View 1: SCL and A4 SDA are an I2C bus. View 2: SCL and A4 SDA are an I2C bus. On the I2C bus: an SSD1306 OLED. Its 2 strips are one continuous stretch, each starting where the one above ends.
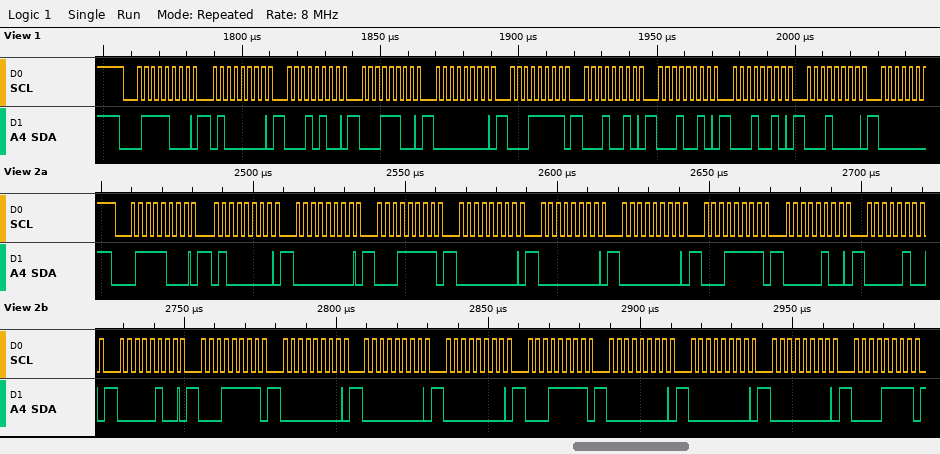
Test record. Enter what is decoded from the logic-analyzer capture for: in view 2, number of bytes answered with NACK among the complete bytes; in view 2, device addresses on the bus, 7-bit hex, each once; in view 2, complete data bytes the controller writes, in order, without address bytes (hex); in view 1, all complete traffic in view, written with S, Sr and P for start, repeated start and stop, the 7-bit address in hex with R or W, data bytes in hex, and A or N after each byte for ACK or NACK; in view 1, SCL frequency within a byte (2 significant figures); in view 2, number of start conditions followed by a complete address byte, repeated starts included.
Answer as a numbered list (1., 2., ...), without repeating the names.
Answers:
1. 0
2. 0x3C
3. 40 00 1F 00 00 00 1F 04 04 04 1F 00 00 00 1F 00 00 00 0F
4. S 3CW A 40 A 14 A 1C A 00 A 1F A 12 A 12 A 12 A 10 A
5. 400 kHz
6. 1
